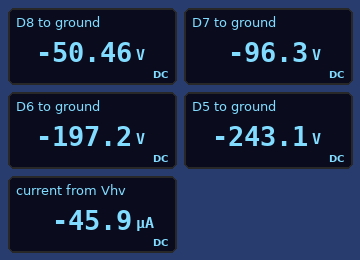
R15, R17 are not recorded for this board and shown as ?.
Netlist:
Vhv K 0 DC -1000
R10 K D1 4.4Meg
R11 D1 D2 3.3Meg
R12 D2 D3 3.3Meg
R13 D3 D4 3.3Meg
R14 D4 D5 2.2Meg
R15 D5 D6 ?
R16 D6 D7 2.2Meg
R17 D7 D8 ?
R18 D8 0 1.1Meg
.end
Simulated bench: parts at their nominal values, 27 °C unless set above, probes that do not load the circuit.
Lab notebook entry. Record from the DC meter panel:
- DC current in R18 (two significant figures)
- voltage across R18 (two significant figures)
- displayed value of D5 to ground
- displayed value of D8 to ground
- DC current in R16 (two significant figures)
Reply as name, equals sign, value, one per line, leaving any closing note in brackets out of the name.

DC current in R18 = 46 µA
voltage across R18 = 50 V
displayed value of D5 to ground = -243.1 V
displayed value of D8 to ground = -50.46 V
DC current in R16 = 46 µA
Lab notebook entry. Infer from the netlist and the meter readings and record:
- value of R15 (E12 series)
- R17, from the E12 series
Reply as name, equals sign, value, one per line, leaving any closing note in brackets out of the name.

value of R15 = 1 MΩ
R17, from the E12 series = 1 MΩ
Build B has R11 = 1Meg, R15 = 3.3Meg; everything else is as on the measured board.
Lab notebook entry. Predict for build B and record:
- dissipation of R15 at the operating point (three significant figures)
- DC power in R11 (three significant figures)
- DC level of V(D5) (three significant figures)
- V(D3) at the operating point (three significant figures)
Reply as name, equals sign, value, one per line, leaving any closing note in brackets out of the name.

dissipation of R15 at the operating point = 6.94 mW
DC power in R11 = 2.10 mW
DC level of V(D5) = -349 V
V(D3) at the operating point = -601 V
